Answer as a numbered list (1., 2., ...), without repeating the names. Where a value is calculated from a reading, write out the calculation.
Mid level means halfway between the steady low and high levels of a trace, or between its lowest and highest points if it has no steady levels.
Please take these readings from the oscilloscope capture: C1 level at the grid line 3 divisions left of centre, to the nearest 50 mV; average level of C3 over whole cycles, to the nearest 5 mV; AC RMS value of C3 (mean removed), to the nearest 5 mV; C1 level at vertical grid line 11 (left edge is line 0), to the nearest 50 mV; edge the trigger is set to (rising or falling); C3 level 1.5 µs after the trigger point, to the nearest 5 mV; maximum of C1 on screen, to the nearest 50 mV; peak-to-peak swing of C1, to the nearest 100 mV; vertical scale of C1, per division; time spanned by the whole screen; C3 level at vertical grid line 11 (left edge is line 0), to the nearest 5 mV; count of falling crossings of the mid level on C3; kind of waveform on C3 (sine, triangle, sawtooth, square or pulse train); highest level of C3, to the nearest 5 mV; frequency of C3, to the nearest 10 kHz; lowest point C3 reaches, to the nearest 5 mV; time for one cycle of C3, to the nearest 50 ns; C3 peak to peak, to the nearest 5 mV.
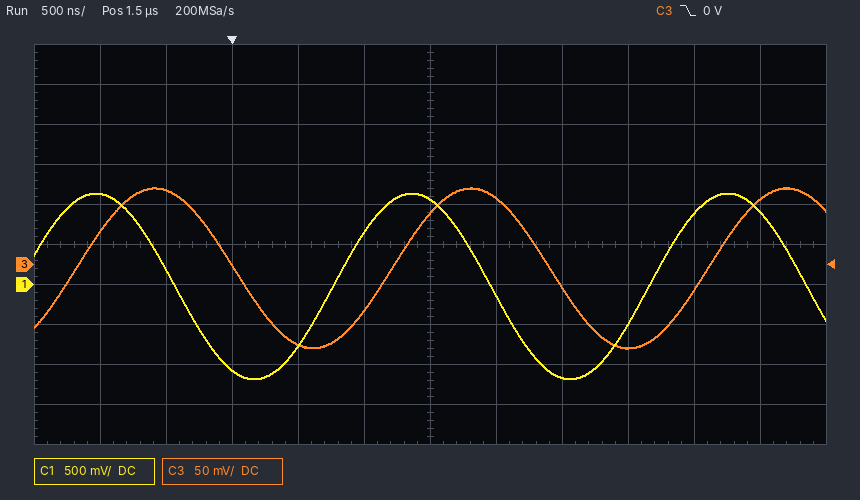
1. -1.05 V
2. (95 mV + (-105 mV)) / 2 ≈ -5 mV
3. 200 mV / (2√2) ≈ 70.7 mV, so 70 mV to the nearest 5 mV
4. 900 mV
5. falling
6. 65 mV
7. 1.15 V
8. 2.30 V
9. 500 mV
10. 6 µs
11. 80 mV
12. 2
13. sine
14. 95 mV
15. 1 / 2.40 µs ≈ 417 kHz, so 420 kHz to the nearest 10 kHz
16. -105 mV
17. 2.40 µs
18. 95 mV − (-105 mV) = 200 mV
